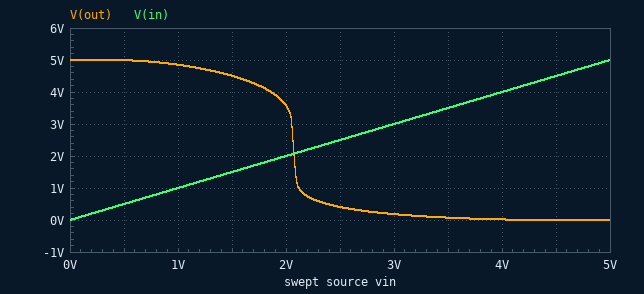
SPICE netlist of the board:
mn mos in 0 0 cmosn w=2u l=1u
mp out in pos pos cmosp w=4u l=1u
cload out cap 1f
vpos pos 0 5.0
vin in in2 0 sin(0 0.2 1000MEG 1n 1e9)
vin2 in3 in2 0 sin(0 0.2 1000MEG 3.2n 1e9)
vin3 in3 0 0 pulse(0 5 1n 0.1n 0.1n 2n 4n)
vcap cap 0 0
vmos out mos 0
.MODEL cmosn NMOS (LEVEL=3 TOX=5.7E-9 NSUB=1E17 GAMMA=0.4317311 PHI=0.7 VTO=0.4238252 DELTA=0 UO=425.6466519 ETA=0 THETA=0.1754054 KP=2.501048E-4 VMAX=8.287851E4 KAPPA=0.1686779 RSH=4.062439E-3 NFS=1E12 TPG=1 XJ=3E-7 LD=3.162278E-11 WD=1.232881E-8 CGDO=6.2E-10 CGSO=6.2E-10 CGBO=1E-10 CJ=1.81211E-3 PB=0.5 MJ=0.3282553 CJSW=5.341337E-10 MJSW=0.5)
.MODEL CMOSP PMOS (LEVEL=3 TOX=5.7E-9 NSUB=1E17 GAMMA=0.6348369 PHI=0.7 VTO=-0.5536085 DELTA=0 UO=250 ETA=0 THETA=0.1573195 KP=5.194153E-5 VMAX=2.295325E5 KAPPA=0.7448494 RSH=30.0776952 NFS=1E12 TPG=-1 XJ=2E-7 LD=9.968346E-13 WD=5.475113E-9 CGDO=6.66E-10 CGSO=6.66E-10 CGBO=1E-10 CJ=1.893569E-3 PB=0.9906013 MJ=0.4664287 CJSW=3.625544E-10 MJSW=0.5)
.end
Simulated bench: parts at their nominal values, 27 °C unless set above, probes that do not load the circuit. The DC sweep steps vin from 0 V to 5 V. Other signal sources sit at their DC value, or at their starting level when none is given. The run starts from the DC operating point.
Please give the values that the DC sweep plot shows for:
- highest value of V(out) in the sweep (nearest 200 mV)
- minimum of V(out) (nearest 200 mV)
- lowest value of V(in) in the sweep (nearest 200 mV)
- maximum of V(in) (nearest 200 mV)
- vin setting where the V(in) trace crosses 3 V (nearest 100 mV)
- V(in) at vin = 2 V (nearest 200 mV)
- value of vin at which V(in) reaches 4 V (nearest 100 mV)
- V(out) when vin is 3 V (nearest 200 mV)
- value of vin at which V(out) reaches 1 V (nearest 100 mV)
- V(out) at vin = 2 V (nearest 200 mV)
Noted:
5.0 V
0 V
0 V
5.0 V
3.0 V
2.0 V
4.0 V
200 mV
2.1 V
3.6 V
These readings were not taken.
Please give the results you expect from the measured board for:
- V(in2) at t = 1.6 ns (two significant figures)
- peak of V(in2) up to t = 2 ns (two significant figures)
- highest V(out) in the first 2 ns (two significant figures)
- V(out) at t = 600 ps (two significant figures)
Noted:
5.0 V
5.0 V
5.6 V
5.0 V
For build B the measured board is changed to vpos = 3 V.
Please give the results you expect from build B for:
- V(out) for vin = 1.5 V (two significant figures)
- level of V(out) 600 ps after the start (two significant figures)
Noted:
180 mV
3.0 V
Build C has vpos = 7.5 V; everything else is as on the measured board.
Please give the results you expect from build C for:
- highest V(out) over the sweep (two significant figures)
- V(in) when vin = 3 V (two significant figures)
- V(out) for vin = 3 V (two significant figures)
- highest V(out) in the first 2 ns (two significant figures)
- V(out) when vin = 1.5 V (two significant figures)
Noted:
7.5 V
3.0 V
5.4 V
8.1 V
7.2 V
